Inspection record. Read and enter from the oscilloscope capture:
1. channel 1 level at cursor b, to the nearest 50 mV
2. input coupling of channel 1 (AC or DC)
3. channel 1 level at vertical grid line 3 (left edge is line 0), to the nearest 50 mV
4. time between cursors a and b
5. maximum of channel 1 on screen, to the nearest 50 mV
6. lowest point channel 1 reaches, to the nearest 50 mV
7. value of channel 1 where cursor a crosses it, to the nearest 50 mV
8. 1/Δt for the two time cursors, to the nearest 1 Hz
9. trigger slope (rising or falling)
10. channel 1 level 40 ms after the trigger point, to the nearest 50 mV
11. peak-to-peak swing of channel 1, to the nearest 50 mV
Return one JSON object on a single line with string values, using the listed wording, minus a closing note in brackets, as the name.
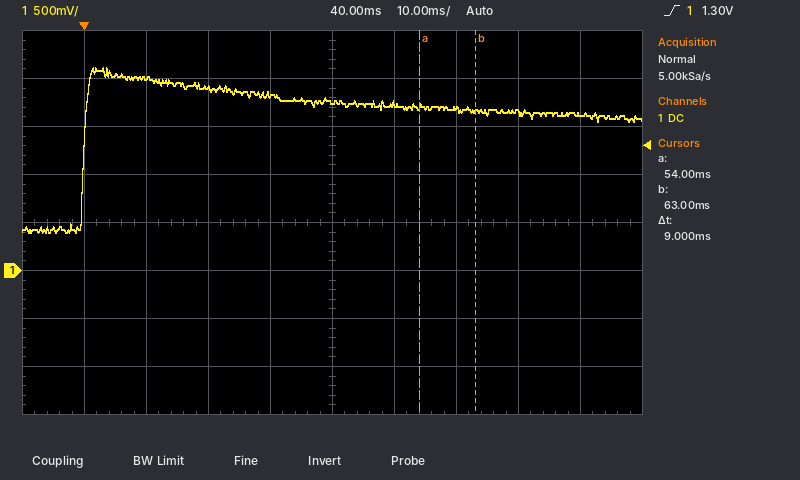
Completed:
{"channel 1 level at cursor b, to the nearest 50 mV": "1.65 V", "input coupling of channel 1": "DC", "channel 1 level at vertical grid line 3 (left edge is line 0), to the nearest 50 mV": "1.90 V", "time between cursors a and b": "9 ms", "maximum of channel 1 on screen, to the nearest 50 mV": "2.10 V", "lowest point channel 1 reaches, to the nearest 50 mV": "400 mV", "value of channel 1 where cursor a crosses it, to the nearest 50 mV": "1.70 V", "1/Δt for the two time cursors, to the nearest 1 Hz": "111 Hz", "trigger slope": "rising", "channel 1 level 40 ms after the trigger point, to the nearest 50 mV": "1.75 V", "peak-to-peak swing of channel 1, to the nearest 50 mV": "1.70 V"}
